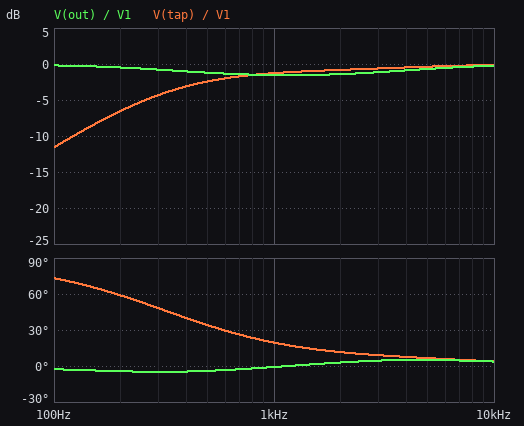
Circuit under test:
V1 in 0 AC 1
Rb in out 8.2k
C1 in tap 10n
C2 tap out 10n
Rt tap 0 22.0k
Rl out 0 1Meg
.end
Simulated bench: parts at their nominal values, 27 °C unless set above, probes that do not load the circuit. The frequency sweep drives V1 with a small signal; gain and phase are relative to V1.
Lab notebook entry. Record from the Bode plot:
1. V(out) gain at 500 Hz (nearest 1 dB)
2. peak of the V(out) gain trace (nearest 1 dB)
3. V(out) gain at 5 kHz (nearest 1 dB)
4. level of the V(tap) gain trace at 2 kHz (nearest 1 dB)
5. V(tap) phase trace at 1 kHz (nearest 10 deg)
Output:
-1 dB
0 dB
-1 dB
-1 dB
20 deg
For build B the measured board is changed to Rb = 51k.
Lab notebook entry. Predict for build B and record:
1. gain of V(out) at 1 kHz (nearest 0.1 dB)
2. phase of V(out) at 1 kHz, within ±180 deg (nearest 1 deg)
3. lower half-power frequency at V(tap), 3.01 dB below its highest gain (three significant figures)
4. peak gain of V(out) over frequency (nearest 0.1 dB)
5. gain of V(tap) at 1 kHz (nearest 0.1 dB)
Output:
-4.0 dB
22 deg
831 Hz
0 dB
-2.5 dB
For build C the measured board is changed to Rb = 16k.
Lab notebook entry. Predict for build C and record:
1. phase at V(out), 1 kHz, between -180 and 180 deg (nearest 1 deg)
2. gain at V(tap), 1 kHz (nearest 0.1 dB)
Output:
2 deg
-1.8 dB
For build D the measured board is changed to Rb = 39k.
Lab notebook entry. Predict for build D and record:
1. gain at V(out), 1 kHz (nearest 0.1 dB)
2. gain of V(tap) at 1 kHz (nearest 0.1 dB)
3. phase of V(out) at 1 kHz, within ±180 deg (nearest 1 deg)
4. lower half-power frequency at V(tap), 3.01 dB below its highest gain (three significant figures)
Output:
-4.0 dB
-2.4 dB
17 deg
789 Hz
